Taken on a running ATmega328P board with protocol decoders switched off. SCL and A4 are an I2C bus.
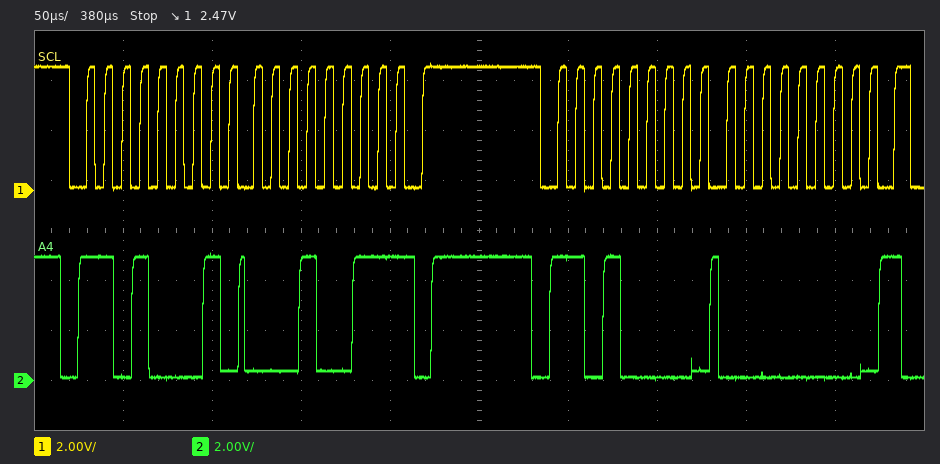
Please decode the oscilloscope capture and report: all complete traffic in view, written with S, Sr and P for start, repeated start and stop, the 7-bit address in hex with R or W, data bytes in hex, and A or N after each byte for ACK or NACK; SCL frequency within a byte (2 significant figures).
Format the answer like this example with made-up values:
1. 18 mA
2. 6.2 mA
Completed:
1. S 68R A 13 N P S 68W A 00 A
2. 100 kHz
